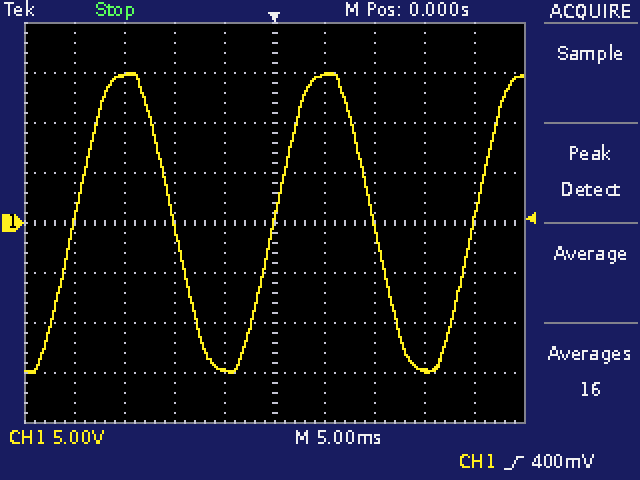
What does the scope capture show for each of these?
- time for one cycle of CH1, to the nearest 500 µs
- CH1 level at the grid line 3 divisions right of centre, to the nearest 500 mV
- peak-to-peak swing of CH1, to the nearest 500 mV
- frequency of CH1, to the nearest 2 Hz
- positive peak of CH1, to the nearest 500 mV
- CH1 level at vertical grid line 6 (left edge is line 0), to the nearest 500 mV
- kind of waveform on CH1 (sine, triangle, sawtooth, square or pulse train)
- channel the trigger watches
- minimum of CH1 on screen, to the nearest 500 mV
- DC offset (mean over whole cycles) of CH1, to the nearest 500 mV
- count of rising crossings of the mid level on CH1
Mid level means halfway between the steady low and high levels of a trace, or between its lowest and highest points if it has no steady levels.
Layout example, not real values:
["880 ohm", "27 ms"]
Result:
["20.0 ms", "-15.0 V", "30.0 V", "50 Hz", "15.0 V", "15.0 V", "sine", "CH1", "-15.0 V", "0.0 V", "3"]
